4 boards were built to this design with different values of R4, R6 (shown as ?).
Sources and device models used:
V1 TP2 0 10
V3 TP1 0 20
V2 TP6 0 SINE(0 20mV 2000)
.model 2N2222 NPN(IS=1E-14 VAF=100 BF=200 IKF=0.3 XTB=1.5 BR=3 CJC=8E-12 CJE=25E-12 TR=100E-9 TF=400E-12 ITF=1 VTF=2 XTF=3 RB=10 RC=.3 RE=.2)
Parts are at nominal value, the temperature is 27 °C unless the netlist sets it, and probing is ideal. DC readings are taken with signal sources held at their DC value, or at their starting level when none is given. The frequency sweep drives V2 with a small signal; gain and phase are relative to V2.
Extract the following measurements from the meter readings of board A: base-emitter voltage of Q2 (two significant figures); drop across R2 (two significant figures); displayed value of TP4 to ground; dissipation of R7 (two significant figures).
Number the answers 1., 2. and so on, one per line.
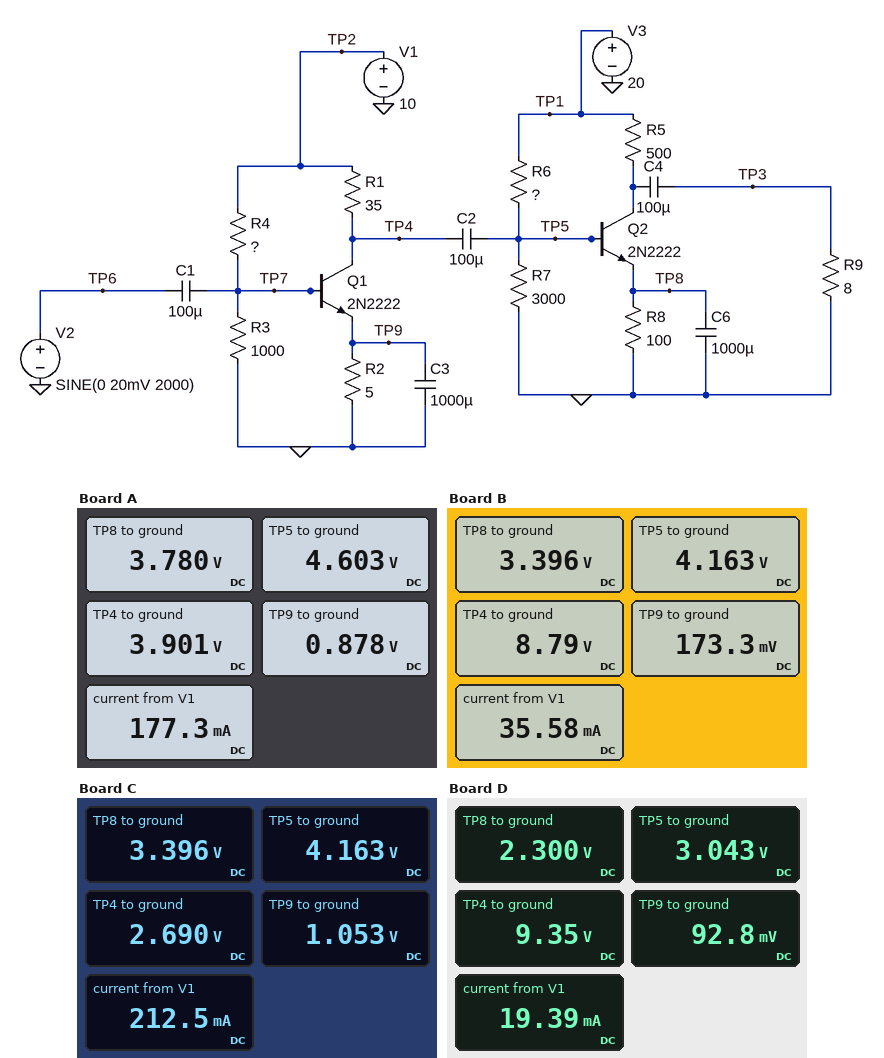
1. 820 mV
2. 880 mV
3. 3.901 V
4. 7.1 mW
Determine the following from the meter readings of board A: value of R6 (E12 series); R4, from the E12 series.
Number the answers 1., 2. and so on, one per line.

1. 2.2 kΩ
2. 2.7 kΩ
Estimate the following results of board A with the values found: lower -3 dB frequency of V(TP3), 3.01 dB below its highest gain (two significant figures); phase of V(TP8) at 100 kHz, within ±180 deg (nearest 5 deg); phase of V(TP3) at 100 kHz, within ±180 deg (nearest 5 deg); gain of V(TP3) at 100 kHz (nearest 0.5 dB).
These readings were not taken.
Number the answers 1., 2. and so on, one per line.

1. 450 Hz
2. 85 deg
3. -15 deg
4. 10.5 dB
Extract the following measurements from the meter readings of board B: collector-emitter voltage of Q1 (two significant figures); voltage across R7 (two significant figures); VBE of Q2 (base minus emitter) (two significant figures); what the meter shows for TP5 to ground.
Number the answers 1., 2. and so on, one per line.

1. 8.6 V
2. 4.2 V
3. 770 mV
4. 4.163 V
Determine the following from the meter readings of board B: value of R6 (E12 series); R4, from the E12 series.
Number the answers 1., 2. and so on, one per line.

1. 6.8 kΩ
2. 8.2 kΩ
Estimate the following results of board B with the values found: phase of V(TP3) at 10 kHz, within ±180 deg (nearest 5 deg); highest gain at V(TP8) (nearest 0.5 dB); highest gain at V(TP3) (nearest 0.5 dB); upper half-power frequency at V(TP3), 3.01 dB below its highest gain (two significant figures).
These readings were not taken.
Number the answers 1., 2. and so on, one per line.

1. 0 deg
2. 1.5 dB
3. 24.5 dB
4. 610 kHz
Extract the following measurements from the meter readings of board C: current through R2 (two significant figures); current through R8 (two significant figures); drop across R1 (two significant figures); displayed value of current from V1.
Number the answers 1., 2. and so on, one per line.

1. 210 mA
2. 34 mA
3. 7.3 V
4. 212.5 mA
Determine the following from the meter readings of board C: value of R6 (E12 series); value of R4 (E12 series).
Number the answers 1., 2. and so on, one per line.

1. 6.8 kΩ
2. 2.2 kΩ
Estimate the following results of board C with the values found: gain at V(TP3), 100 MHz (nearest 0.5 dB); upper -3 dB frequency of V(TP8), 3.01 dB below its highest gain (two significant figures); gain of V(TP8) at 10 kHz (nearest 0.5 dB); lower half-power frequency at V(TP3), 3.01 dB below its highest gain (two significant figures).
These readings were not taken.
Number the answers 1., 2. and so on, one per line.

1. -17.0 dB
2. 670 Hz
3. -20.5 dB
4. 460 Hz
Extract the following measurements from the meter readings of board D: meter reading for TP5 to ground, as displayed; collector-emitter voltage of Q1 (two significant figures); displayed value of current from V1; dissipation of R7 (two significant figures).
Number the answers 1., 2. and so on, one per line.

1. 3.043 V
2. 9.3 V
3. 19.39 mA
4. 3.1 mW
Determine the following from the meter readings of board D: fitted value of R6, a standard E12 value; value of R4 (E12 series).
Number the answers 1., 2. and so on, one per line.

1. 15 kΩ
2. 10 kΩ
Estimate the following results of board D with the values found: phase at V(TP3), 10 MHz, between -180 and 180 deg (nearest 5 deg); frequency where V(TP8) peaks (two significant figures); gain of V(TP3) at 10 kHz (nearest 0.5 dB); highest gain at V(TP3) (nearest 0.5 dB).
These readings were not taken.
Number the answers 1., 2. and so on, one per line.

1. -50 deg
2. 110 Hz
3. 39.5 dB
4. 39.5 dB
